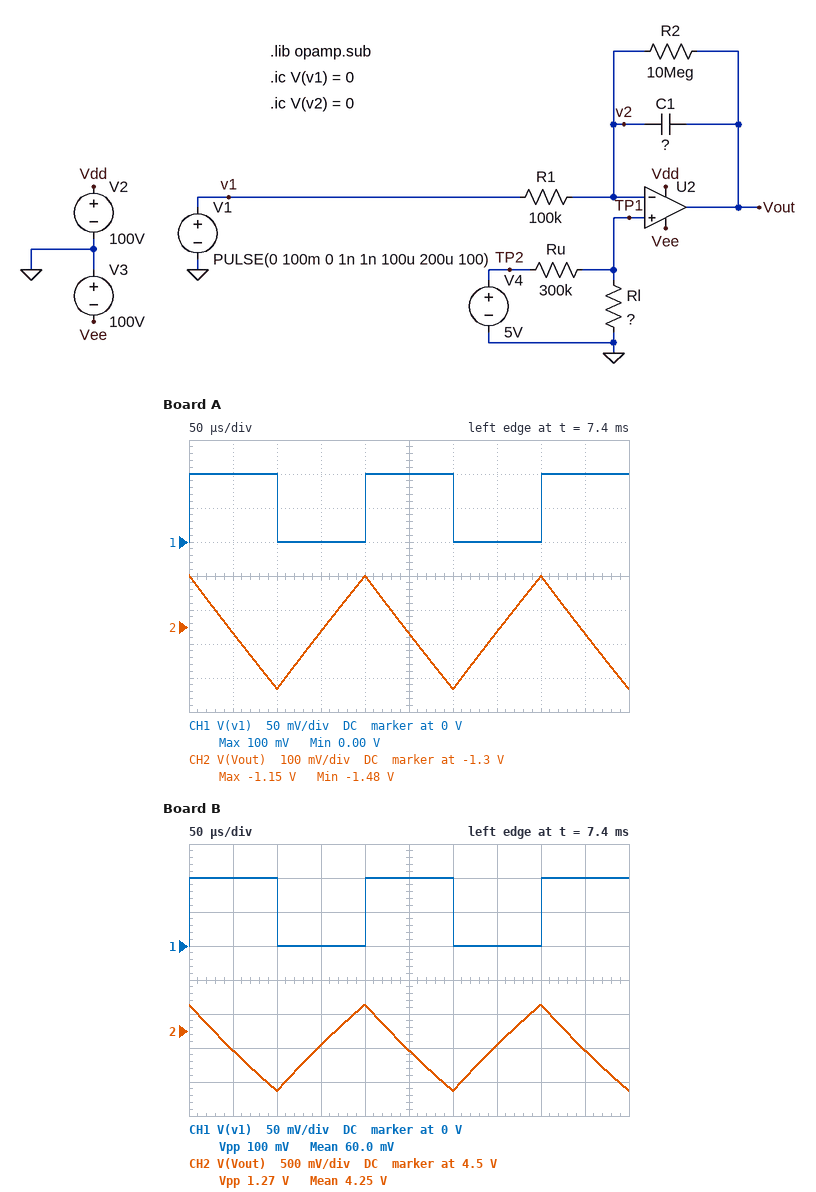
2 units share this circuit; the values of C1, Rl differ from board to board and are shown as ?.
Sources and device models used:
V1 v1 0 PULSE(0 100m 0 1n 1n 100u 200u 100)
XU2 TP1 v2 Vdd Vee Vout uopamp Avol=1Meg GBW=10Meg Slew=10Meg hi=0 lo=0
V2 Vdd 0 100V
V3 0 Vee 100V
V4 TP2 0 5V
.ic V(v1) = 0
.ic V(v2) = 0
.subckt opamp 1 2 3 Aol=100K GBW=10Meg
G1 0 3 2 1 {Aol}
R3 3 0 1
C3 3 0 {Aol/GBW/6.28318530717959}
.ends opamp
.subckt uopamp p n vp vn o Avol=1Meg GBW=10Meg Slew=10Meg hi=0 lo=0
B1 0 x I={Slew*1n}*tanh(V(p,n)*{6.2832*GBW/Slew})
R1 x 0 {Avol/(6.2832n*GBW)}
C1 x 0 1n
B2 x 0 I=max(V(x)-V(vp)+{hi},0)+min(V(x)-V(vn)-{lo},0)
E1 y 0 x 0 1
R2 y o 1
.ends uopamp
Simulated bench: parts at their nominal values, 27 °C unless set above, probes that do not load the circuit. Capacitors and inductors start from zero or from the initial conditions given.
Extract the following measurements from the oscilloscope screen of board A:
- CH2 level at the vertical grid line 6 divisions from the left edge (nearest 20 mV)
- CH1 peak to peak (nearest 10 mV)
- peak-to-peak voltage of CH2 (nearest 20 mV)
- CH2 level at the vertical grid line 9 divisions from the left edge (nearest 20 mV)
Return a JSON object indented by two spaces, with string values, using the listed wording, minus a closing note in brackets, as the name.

{
  "CH2 level at the vertical grid line 6 divisions from the left edge": "-1.48 V",
  "CH1 peak to peak": "100 mV",
  "peak-to-peak voltage of CH2": "340 mV",
  "CH2 level at the vertical grid line 9 divisions from the left edge": "-1.32 V"
}
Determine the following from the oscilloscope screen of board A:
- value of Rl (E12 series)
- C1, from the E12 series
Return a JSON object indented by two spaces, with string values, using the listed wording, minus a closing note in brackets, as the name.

{
  "value of Rl": "2.2 kΩ",
  "C1, from the E12 series": "150 pF"
}
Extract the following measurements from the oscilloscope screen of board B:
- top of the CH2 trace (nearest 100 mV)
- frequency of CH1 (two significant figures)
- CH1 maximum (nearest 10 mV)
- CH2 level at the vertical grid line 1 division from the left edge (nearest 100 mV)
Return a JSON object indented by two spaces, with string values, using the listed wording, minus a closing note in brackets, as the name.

{
  "top of the CH2 trace": "4.9 V",
  "frequency of CH1": "5.0 kHz",
  "CH1 maximum": "100 mV",
  "CH2 level at the vertical grid line 1 division from the left edge": "4.2 V"
}
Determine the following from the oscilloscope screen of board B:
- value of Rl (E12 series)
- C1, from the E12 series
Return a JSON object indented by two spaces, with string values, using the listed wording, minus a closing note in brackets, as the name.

{
  "value of Rl": "5.6 kΩ",
  "C1, from the E12 series": "39 pF"
}
